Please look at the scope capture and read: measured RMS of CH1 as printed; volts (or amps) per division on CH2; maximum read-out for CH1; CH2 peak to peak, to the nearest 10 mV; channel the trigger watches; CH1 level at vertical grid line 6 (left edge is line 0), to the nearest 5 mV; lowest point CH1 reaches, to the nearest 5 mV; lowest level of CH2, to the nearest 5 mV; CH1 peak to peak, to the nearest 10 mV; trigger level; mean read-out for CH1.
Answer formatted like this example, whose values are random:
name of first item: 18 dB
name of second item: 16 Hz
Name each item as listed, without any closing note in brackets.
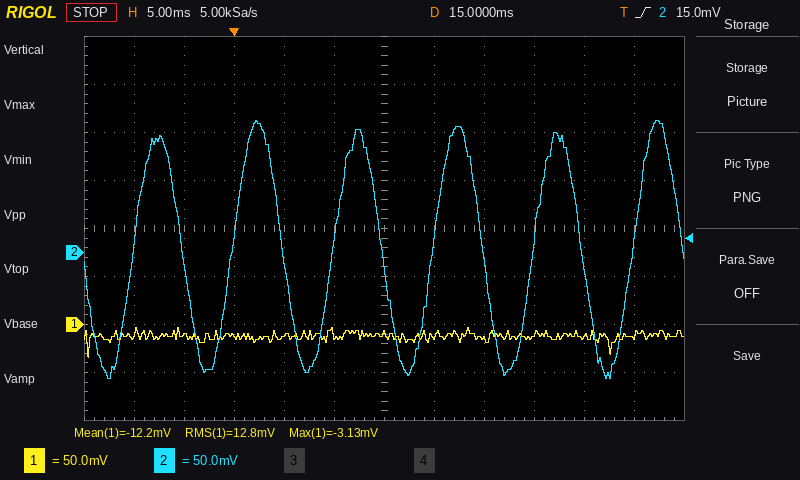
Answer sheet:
measured RMS of CH1 as printed: 12.8 mV
volts (or amps) per division on CH2: 50 mV
maximum read-out for CH1: -3.13 mV
CH2 peak to peak, to the nearest 10 mV: 270 mV
channel the trigger watches: CH2
CH1 level at vertical grid line 6 (left edge is line 0), to the nearest 5 mV: -10 mV
lowest point CH1 reaches, to the nearest 5 mV: -35 mV
lowest level of CH2, to the nearest 5 mV: -130 mV
CH1 peak to peak, to the nearest 10 mV: 30 mV
trigger level: 15.0 mV
mean read-out for CH1: -12.2 mV
